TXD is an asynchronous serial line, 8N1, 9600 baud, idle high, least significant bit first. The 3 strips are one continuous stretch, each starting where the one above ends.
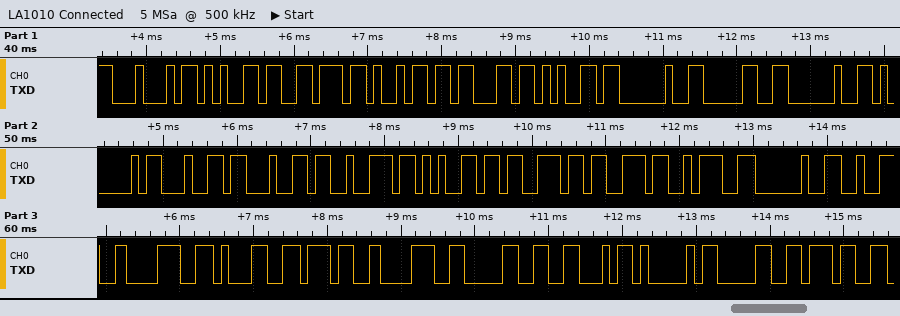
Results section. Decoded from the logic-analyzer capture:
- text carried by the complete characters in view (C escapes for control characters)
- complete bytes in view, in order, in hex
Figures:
"Device 0 Address: 281780FA07"
44 65 76 69 63 65 20 30 20 41 64 64 72 65 73 73 3A 20 32 38 31 37 38 30 46 41 30 37
